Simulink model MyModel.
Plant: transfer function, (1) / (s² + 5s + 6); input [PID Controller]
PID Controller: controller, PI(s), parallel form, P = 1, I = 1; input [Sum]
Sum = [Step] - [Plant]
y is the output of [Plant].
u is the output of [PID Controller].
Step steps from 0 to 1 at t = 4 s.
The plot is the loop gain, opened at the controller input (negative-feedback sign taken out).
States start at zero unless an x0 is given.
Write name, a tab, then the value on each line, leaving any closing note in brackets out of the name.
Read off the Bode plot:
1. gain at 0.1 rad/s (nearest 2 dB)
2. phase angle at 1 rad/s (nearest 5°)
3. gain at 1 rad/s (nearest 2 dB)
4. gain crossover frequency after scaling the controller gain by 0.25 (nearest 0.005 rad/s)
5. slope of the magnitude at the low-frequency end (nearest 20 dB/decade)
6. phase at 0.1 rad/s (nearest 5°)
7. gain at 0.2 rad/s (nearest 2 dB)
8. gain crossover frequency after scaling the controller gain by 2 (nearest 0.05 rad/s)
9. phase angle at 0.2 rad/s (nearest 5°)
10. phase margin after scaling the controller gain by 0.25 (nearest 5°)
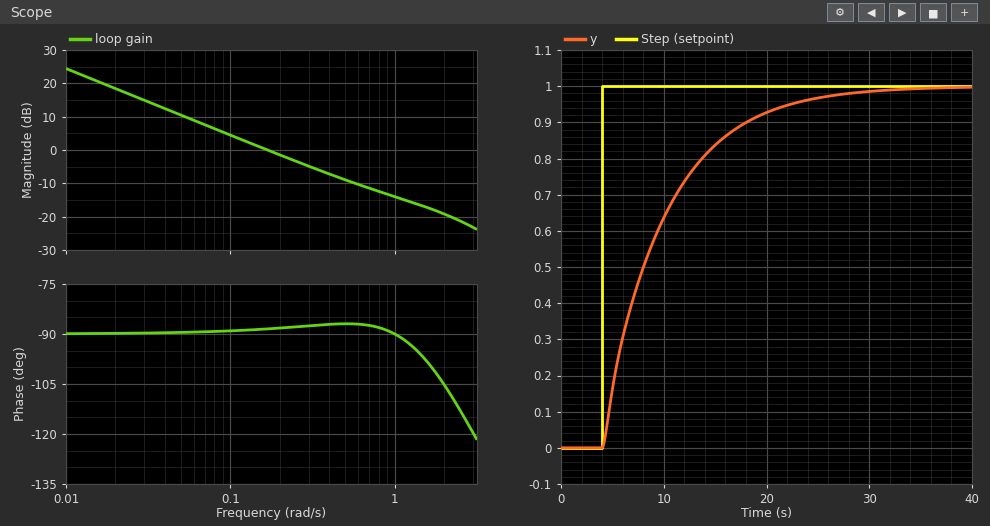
gain at 0.1 rad/s	4 dB
phase angle at 1 rad/s	-90°
gain at 1 rad/s	-14 dB
gain crossover frequency after scaling the controller gain by 0.25	0.040 rad/s
slope of the magnitude at the low-frequency end	-20 dB/decade
phase at 0.1 rad/s	-90°
gain at 0.2 rad/s	-2 dB
gain crossover frequency after scaling the controller gain by 2	0.35 rad/s
phase angle at 0.2 rad/s	-90°
phase margin after scaling the controller gain by 0.25	90°
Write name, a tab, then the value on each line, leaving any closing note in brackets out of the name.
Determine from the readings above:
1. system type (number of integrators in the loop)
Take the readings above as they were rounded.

system type	1
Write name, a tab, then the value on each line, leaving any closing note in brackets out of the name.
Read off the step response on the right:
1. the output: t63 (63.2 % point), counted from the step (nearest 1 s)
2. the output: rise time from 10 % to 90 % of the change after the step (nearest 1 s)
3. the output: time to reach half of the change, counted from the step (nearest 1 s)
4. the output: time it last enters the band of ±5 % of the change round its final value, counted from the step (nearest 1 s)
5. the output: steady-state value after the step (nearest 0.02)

the output: t63 (63.2 % point), counted from the step	6 s
the output: rise time from 10 % to 90 % of the change after the step	13 s
the output: time to reach half of the change, counted from the step	4 s
the output: time it last enters the band of ±5 % of the change round its final value, counted from the step	18 s
the output: steady-state value after the step	1.00
